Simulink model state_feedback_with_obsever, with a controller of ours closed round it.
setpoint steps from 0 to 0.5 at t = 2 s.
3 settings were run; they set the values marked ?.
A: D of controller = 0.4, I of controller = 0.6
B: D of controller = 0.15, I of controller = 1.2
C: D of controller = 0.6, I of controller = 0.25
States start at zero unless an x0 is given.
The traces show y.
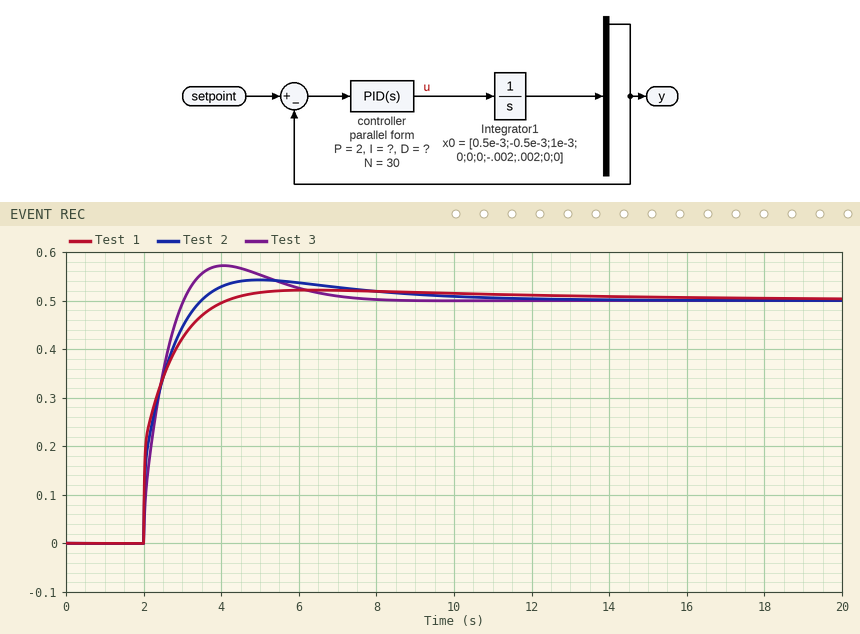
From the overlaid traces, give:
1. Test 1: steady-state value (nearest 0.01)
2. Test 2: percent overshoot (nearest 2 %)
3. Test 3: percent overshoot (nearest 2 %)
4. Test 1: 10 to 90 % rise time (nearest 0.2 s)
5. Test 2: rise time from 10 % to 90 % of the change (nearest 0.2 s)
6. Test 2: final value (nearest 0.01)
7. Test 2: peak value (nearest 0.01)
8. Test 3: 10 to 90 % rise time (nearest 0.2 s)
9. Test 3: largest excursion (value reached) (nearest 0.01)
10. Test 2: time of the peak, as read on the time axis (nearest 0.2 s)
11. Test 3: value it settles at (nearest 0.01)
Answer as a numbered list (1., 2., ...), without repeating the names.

1. 0.50
2. 8 %
3. 14 %
4. 1.2 s
5. 1.0 s
6. 0.50
7. 0.54
8. 0.8 s
9. 0.57
10. 5.0 s
11. 0.50
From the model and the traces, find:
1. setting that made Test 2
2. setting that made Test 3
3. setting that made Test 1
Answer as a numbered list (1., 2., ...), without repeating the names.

1. A
2. B
3. C
